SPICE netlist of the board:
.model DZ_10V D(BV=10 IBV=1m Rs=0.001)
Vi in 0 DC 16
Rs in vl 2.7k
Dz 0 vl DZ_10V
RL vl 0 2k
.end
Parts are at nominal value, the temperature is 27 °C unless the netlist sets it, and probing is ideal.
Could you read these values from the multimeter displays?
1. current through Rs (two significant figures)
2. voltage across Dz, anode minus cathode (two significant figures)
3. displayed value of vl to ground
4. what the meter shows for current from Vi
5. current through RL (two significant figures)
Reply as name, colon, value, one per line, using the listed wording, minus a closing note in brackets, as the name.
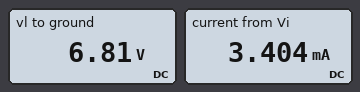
current through Rs: 3.4 mA
voltage across Dz, anode minus cathode: -6.8 V
displayed value of vl to ground: 6.81 V
what the meter shows for current from Vi: 3.404 mA
current through RL: 3.4 mA
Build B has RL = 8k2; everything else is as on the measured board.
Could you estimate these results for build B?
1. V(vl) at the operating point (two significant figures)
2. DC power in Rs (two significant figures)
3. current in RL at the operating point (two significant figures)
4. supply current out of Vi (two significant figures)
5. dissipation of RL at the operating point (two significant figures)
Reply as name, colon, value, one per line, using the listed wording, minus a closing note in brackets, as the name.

V(vl) at the operating point: 10 V
DC power in Rs: 13 mW
current in RL at the operating point: 1.2 mA
supply current out of Vi: 2.2 mA
dissipation of RL at the operating point: 12 mW
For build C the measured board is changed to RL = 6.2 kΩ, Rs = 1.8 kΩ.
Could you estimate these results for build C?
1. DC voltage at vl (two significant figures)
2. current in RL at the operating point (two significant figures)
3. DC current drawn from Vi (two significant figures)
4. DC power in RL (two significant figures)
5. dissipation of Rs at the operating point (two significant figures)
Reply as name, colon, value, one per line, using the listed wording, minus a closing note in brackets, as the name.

DC voltage at vl: 10 V
current in RL at the operating point: 1.6 mA
DC current drawn from Vi: 3.3 mA
DC power in RL: 16 mW
dissipation of Rs at the operating point: 20 mW
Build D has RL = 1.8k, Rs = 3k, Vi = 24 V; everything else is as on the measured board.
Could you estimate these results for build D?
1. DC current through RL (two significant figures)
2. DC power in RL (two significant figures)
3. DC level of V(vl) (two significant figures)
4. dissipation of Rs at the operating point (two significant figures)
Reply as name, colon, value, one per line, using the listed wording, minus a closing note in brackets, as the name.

DC current through RL: 5.0 mA
DC power in RL: 45 mW
DC level of V(vl): 9.0 V
dissipation of Rs at the operating point: 75 mW
